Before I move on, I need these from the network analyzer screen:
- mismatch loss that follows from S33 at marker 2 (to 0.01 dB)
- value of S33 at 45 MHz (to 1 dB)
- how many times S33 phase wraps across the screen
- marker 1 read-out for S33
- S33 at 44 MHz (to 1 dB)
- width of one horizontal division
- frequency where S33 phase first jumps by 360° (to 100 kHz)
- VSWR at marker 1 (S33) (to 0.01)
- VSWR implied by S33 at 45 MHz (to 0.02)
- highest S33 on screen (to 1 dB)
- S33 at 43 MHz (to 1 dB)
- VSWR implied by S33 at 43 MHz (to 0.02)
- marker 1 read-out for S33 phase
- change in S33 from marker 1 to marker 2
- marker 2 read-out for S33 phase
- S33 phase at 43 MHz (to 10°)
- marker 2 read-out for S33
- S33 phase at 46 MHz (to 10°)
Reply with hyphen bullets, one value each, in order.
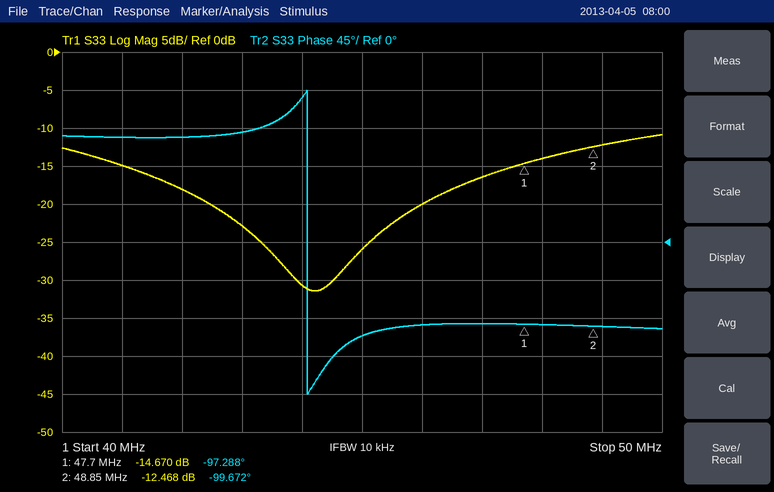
- 0.25 dB
- -26 dB
- 1
- -14.670 dB
- -31 dB
- 1 MHz
- 44.1 MHz
- 1.45
- 1.10
- -11 dB
- -23 dB
- 1.16
- -97.288°
- 2.202 dB
- -99.672°
- 130°
- -12.468 dB
- -100°
